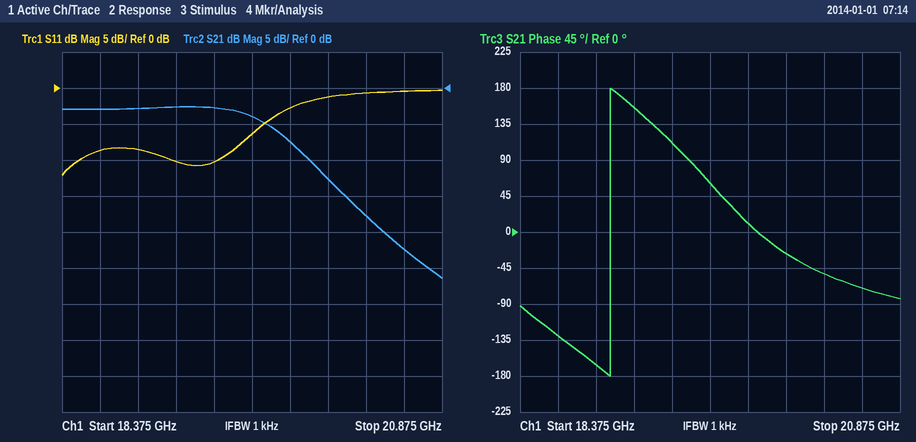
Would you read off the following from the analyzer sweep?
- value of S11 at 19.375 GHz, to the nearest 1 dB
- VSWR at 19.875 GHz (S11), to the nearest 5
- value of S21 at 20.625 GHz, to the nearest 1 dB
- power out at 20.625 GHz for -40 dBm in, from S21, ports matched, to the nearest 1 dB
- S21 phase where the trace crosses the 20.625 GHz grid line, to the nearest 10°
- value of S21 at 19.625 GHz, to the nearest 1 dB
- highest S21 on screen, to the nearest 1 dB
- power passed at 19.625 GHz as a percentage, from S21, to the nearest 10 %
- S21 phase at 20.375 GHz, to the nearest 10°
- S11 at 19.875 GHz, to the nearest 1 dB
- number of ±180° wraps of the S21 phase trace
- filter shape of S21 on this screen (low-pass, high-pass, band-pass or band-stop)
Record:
-10 dB
5
-22 dB
-62 dBm
-70°
-4 dB
-3 dB
40 %
-50°
-3 dB
1
low-pass
